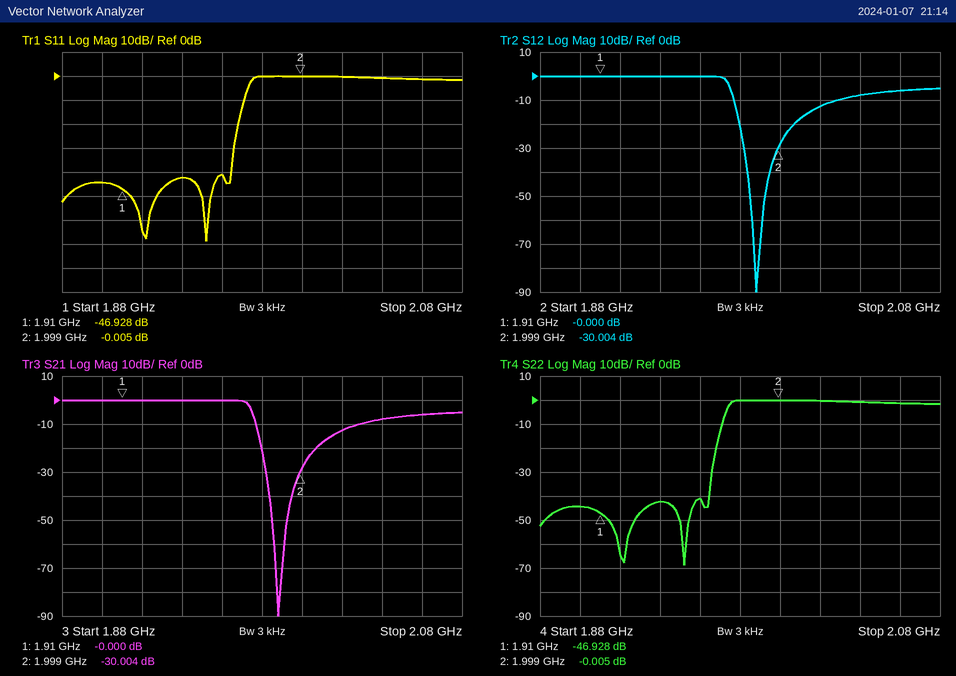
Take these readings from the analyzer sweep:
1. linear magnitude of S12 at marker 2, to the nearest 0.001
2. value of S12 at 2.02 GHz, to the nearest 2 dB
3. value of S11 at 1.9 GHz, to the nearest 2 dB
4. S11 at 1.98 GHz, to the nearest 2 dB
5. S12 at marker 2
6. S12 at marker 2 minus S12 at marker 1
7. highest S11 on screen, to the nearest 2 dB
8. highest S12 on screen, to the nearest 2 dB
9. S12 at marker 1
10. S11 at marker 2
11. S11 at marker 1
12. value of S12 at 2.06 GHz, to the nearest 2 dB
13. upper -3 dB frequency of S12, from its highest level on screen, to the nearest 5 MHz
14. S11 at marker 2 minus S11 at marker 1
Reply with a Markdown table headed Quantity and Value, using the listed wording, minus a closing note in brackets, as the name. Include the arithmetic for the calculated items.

| Quantity | Value |
|---|---|
| linear magnitude of S12 at marker 2, to the nearest 0.001 | 10^(-30.004/20) ≈ 0.032 |
| value of S12 at 2.02 GHz, to the nearest 2 dB | -12 dB |
| value of S11 at 1.9 GHz, to the nearest 2 dB | -44 dB |
| S11 at 1.98 GHz, to the nearest 2 dB | 0 dB |
| S12 at marker 2 | -30.004 dB |
| S12 at marker 2 minus S12 at marker 1 | -30.004 − (-0) = -30.004 dB |
| highest S11 on screen, to the nearest 2 dB | 0 dB |
| highest S12 on screen, to the nearest 2 dB | 0 dB |
| S12 at marker 1 | -0.000 dB |
| S11 at marker 2 | -0.005 dB |
| S11 at marker 1 | -46.928 dB |
| value of S12 at 2.06 GHz, to the nearest 2 dB | -6 dB |
| upper -3 dB frequency of S12, from its highest level on screen, to the nearest 5 MHz | 1.975 GHz |
| S11 at marker 2 minus S11 at marker 1 | -0.005 − (-46.928) = 46.923 dB |
